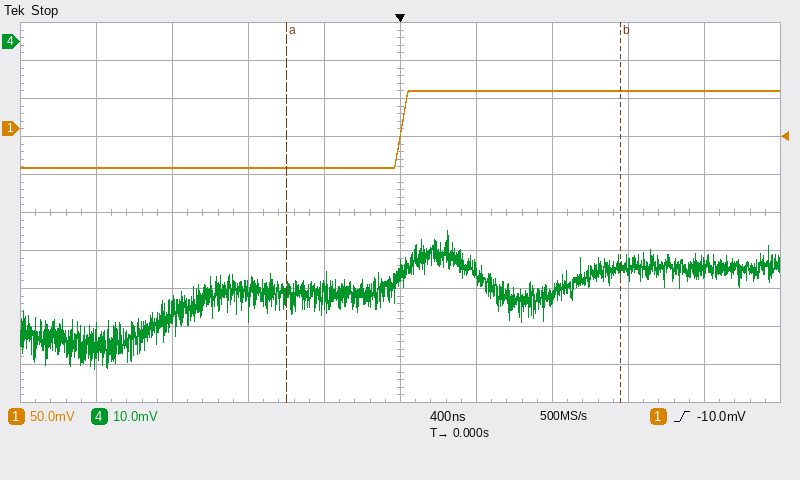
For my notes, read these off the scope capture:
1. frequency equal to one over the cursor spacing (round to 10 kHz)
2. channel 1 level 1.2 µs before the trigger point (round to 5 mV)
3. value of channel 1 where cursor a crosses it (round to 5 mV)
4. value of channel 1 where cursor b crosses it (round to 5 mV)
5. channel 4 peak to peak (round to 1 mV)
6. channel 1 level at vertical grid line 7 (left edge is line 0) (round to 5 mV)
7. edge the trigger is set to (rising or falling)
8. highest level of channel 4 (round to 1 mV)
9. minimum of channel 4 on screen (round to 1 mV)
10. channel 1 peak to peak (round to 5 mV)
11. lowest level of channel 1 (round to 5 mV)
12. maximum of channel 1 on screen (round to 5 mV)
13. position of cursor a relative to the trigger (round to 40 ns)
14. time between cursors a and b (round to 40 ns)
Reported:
570 kHz
-50 mV
-50 mV
50 mV
36 mV
50 mV
rising
-50 mV
-86 mV
100 mV
-50 mV
50 mV
-600 ns
1.76 µs
